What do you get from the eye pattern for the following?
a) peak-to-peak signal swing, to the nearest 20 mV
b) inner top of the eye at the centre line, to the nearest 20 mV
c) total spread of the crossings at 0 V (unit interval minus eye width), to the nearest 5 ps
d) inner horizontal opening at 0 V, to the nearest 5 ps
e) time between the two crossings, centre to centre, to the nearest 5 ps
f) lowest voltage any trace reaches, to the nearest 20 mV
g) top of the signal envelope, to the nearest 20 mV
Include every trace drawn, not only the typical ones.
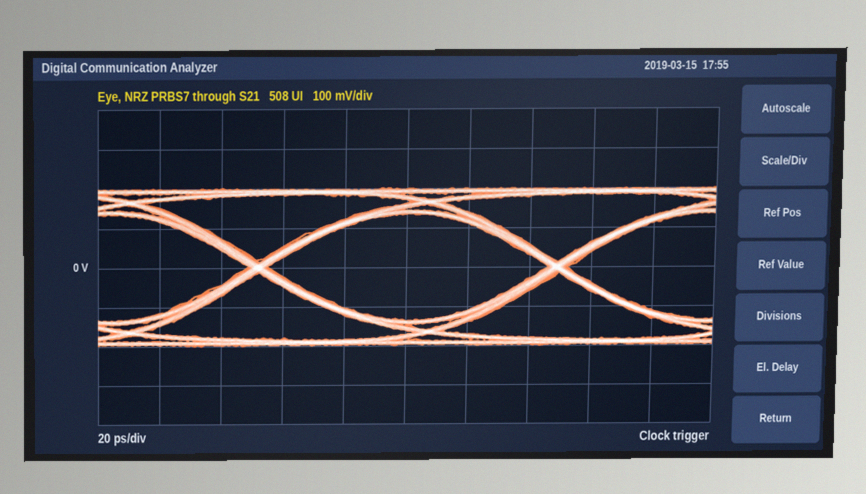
400 mV
140 mV
5 ps
90 ps
95 ps
-200 mV
200 mV
